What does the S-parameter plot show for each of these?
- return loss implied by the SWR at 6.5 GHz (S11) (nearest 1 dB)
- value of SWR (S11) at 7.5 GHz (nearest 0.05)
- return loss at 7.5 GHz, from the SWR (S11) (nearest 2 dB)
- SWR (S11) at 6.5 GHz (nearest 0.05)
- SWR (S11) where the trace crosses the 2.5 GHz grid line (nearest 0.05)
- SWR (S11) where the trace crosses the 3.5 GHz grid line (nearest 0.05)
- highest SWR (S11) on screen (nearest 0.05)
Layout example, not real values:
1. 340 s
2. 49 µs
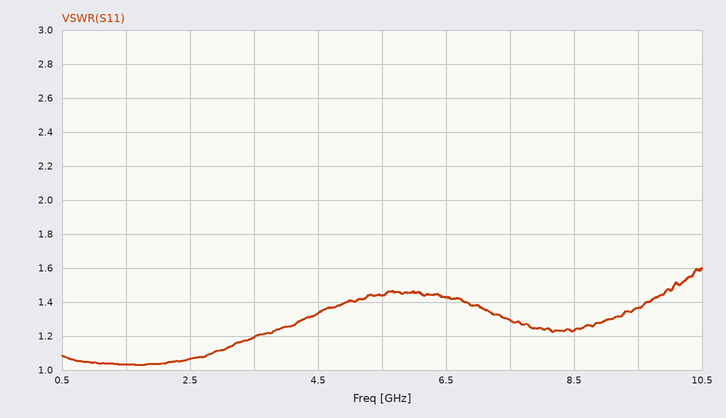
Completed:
1. 15 dB
2. 1.30
3. 18 dB
4. 1.45
5. 1.05
6. 1.20
7. 1.60
